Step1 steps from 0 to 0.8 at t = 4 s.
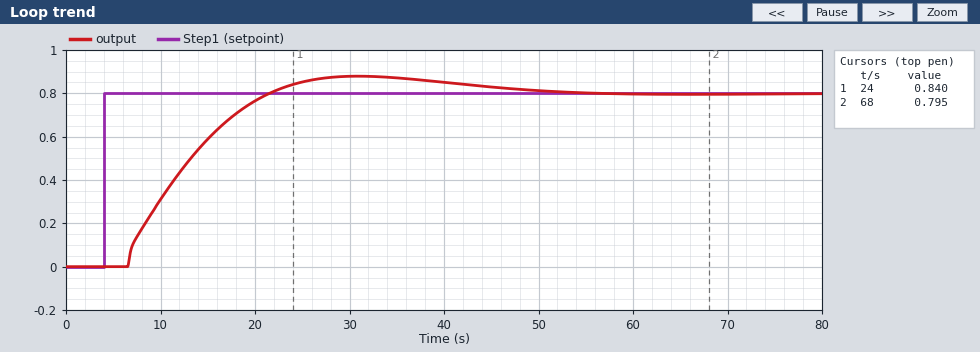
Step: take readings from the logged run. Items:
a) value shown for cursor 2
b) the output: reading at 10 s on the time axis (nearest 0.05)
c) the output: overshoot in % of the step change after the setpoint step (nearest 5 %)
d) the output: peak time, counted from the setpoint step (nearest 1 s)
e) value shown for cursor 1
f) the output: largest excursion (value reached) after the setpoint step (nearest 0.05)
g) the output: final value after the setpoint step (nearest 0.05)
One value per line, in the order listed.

0.795
0.30
10 %
27 s
0.840
0.90
0.80
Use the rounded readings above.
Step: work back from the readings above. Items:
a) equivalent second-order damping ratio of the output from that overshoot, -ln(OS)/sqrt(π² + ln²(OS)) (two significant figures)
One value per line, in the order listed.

0.59
